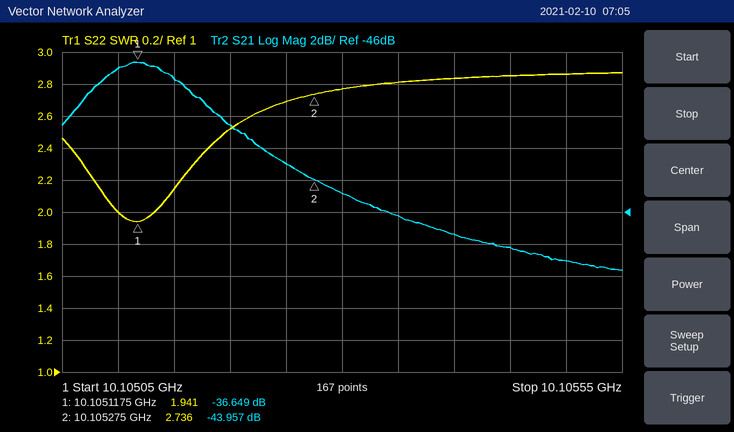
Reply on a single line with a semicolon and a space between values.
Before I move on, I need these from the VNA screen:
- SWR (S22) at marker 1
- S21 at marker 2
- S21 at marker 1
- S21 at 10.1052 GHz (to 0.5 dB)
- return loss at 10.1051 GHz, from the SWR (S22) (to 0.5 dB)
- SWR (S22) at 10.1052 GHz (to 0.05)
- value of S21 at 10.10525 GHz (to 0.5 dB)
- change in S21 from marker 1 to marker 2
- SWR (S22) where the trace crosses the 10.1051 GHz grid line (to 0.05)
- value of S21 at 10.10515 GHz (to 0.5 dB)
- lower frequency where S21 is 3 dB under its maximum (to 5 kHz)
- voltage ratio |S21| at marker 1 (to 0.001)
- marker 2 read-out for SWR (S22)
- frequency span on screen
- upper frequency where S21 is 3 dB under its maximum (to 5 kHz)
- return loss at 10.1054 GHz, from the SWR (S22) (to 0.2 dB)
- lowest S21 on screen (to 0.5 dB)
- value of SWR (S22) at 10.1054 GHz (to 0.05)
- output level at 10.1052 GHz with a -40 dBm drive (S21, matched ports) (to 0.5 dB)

1.941; -43.957 dB; -36.649 dB; -40.5 dB; 9.5 dB; 2.50; -43.0 dB; -7.308 dB; 2.00; -37.5 dB; 10.105060 GHz; 0.015; 2.736; 500 kHz; 10.105185 GHz; 6.4 dB; -49.5 dB; 2.85; -80.5 dBm
